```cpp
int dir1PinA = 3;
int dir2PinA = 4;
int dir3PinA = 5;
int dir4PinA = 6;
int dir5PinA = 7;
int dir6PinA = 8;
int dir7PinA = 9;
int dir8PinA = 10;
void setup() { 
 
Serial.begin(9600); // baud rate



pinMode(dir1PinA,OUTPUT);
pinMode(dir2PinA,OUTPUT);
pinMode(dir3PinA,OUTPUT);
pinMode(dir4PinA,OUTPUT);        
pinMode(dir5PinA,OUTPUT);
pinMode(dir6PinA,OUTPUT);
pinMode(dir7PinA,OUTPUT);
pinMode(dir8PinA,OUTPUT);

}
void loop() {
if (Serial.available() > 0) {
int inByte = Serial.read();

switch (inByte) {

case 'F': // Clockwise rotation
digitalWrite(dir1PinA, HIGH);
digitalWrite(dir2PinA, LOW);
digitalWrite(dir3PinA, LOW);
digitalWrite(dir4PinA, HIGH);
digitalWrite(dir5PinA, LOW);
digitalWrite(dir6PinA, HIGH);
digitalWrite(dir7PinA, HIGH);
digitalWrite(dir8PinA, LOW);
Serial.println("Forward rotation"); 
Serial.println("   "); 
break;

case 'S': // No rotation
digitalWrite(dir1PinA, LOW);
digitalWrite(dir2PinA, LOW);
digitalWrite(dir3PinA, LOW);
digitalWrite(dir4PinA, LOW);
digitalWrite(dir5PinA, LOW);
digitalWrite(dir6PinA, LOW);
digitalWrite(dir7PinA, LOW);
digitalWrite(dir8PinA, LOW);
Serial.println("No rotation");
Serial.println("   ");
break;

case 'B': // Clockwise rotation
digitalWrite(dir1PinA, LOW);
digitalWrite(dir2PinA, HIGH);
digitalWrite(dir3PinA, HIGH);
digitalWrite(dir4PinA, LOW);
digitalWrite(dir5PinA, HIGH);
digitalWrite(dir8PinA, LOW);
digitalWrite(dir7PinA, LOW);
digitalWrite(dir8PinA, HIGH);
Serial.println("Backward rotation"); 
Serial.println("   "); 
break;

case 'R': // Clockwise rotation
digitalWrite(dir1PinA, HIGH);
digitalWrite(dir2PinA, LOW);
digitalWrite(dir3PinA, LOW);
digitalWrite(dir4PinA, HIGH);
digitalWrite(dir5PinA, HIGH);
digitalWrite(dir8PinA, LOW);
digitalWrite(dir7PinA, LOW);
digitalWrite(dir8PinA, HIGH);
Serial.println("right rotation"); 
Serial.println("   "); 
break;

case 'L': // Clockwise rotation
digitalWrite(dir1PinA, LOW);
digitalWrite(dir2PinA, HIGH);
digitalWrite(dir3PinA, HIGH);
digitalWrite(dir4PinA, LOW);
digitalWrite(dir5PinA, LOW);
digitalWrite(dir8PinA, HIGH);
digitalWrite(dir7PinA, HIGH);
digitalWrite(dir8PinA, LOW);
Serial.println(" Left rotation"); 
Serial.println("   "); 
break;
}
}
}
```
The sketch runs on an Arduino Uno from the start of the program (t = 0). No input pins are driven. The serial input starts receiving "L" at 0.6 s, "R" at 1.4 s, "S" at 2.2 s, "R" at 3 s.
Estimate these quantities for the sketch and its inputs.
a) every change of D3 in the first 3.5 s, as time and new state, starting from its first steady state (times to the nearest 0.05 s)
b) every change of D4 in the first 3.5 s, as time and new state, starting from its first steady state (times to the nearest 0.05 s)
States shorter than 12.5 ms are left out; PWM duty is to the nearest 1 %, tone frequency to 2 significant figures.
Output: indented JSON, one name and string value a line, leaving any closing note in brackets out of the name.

{
  "every change of D3 in the first 3.5 s, as time and new state, starting from its first steady state": "0 s low; 1.4 s high; 2.2 s low; 3 s high",
  "every change of D4 in the first 3.5 s, as time and new state, starting from its first steady state": "0 s low; 0.6 s high; 1.4 s low"
}
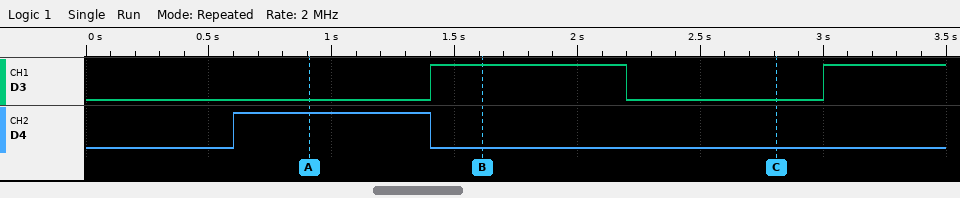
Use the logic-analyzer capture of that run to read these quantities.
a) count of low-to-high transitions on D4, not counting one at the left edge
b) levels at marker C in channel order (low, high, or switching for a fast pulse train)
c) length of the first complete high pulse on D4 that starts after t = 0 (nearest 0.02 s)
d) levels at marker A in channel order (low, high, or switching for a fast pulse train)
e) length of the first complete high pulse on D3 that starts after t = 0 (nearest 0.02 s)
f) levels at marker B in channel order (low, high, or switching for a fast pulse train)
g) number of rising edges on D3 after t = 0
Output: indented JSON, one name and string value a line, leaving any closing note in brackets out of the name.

{
  "count of low-to-high transitions on D4, not counting one at the left edge": "1",
  "levels at marker C in channel order": "D3 low, D4 low",
  "length of the first complete high pulse on D4 that starts after t = 0": "0.80 s",
  "levels at marker A in channel order": "D3 low, D4 high",
  "length of the first complete high pulse on D3 that starts after t = 0": "0.80 s",
  "levels at marker B in channel order": "D3 high, D4 low",
  "number of rising edges on D3 after t = 0": "2"
}
